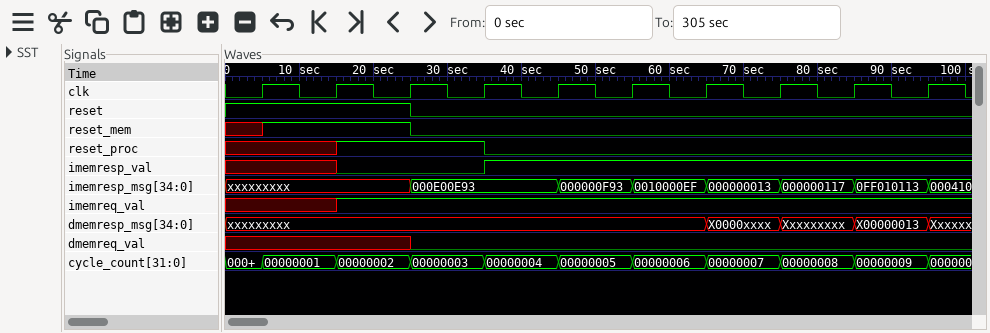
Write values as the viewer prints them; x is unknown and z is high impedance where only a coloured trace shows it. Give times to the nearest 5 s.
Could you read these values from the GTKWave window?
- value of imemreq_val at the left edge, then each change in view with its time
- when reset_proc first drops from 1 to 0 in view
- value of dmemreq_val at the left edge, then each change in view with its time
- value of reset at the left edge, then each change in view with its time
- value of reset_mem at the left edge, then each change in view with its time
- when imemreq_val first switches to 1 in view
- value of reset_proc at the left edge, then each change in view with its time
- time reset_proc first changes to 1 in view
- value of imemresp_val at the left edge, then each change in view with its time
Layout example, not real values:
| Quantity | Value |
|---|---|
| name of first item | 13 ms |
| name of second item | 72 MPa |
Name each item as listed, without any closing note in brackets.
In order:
| Quantity | Value |
|---|---|
| value of imemreq_val at the left edge, then each change in view with its time | x, 1 at 15 s |
| when reset_proc first drops from 1 to 0 in view | 35 s |
| value of dmemreq_val at the left edge, then each change in view with its time | x, 0 at 25 s |
| value of reset at the left edge, then each change in view with its time | 1, 0 at 25 s |
| value of reset_mem at the left edge, then each change in view with its time | x, 1 at 5 s, 0 at 25 s |
| when imemreq_val first switches to 1 in view | 15 s |
| value of reset_proc at the left edge, then each change in view with its time | x, 1 at 15 s, 0 at 35 s |
| time reset_proc first changes to 1 in view | 15 s |
| value of imemresp_val at the left edge, then each change in view with its time | x, 0 at 15 s, 1 at 35 s |
